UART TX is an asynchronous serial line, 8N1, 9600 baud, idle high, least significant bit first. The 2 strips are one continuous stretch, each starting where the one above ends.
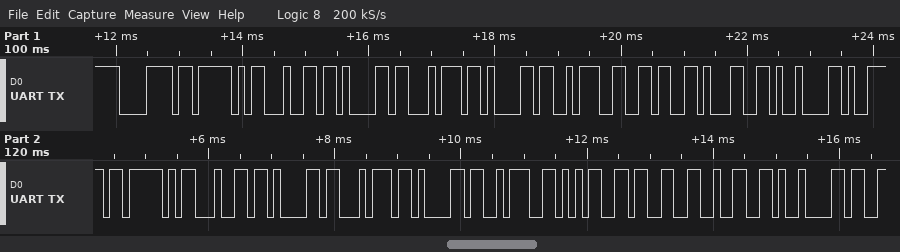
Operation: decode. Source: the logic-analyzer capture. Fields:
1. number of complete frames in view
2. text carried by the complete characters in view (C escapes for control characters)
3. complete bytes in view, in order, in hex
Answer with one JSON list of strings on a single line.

["21", "\"x_data:61\\ty_data:532\\t\"", "78 5F 64 61 74 61 3A 36 31 09 79 5F 64 61 74 61 3A 35 33 32 09"]
